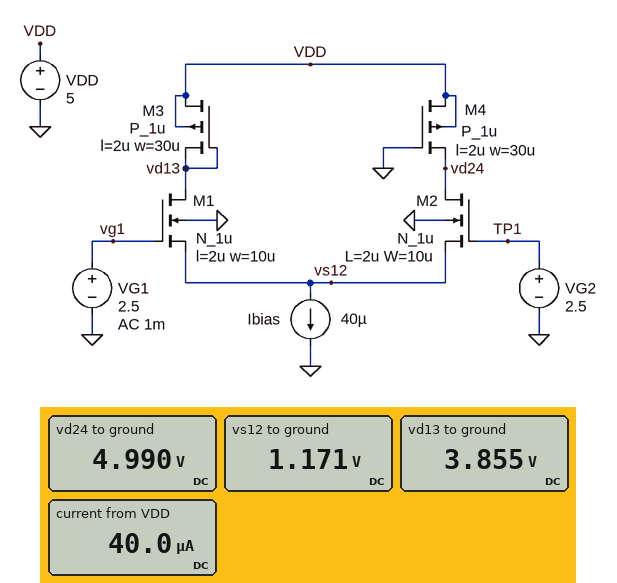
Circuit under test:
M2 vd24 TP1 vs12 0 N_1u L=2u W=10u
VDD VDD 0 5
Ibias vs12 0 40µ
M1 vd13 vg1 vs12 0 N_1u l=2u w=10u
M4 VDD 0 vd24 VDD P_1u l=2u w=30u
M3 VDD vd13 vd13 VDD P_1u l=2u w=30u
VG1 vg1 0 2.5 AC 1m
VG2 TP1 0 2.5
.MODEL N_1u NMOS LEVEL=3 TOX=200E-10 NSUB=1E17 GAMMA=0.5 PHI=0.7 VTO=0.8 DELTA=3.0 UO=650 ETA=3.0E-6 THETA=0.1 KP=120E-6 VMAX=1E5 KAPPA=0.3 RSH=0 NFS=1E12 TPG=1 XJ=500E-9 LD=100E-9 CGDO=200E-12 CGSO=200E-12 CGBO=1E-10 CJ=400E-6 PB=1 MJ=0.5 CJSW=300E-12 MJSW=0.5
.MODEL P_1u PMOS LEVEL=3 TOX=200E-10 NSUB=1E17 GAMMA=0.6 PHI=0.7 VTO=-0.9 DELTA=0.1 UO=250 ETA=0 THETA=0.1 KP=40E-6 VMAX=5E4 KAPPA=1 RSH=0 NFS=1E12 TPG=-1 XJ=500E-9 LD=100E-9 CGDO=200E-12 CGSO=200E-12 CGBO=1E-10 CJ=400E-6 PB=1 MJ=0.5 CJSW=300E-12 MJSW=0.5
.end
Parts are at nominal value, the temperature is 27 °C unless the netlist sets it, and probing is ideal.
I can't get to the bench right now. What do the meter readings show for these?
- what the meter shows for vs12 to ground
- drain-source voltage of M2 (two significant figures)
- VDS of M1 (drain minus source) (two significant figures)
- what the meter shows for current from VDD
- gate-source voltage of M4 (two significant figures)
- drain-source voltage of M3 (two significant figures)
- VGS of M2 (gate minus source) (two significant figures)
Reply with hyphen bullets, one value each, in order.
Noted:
- 1.171 V
- 3.8 V
- 2.7 V
- 40.0 µA
- -5.0 V
- 1.1 V
- 1.3 V
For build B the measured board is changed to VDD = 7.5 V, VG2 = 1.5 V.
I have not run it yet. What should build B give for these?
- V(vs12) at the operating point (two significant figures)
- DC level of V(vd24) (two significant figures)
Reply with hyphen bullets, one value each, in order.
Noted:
- 1.1 V
- 7.5 V
